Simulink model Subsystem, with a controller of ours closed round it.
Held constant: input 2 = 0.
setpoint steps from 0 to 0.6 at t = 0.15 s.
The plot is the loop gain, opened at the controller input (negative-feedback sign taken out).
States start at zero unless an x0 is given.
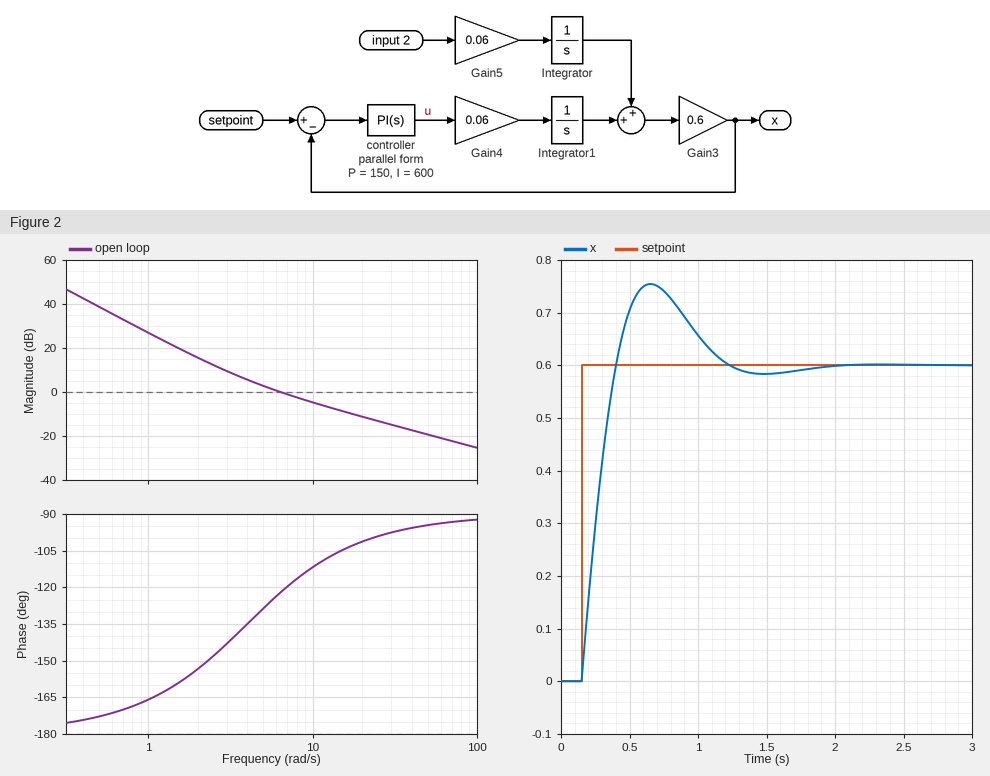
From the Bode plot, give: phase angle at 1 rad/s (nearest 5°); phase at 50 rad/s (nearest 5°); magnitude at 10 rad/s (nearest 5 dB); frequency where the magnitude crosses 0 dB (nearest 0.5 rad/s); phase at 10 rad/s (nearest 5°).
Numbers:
-165°
-95°
-5 dB
6.5 rad/s
-110°
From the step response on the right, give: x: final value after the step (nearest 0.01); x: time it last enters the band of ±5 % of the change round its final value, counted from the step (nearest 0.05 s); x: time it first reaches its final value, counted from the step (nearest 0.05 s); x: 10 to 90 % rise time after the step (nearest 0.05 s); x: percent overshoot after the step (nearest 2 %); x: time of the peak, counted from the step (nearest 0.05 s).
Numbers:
0.60
0.95 s
0.25 s
0.20 s
26 %
0.50 s
